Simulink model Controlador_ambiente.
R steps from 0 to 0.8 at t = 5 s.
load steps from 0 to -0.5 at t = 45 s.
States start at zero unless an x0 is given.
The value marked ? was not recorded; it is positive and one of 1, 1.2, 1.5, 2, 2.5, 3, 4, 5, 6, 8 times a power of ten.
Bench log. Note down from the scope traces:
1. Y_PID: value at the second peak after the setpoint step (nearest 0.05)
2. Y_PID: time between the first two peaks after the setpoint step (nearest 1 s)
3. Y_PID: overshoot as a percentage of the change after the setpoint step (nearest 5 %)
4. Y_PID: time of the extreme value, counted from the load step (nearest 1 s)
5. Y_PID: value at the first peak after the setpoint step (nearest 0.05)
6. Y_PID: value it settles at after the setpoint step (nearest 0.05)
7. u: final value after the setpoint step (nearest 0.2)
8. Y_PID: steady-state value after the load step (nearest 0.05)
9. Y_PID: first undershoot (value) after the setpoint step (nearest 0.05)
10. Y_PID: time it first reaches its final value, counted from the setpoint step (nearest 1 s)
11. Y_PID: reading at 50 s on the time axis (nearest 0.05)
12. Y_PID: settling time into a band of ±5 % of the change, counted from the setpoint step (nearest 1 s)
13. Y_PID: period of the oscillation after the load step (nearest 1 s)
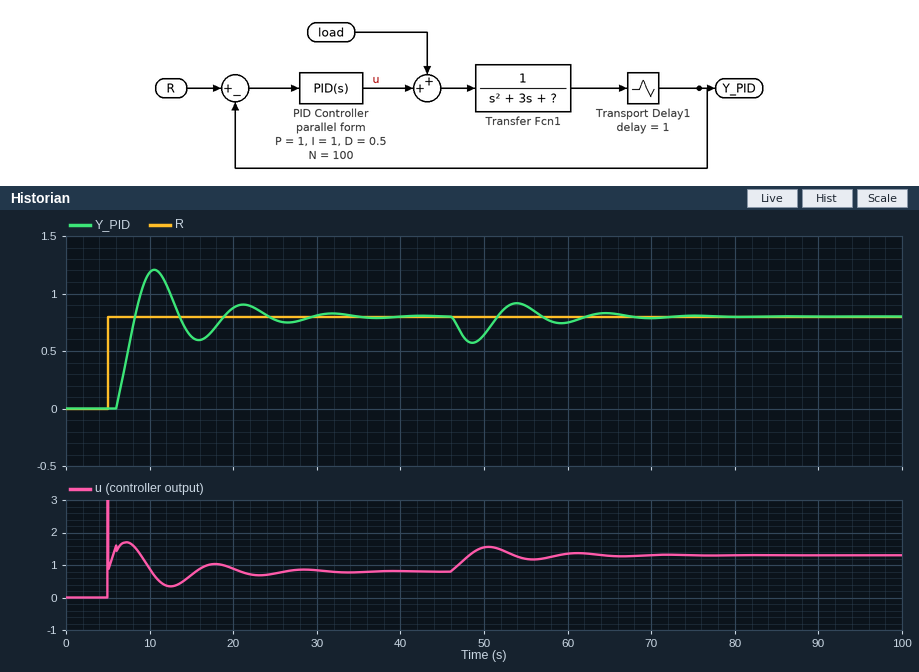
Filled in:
0.90
11 s
50 %
4 s
1.20
0.80
0.8
0.80
0.60
3 s
0.65
23 s
11 s
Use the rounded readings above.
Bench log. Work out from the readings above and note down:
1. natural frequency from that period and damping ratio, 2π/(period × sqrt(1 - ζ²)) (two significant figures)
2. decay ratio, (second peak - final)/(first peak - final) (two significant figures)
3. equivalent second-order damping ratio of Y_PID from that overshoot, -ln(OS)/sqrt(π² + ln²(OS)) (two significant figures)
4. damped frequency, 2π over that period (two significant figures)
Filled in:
0.59 rad/s
0.25
0.22
0.57 rad/s
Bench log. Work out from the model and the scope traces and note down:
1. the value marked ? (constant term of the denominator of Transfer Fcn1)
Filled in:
1
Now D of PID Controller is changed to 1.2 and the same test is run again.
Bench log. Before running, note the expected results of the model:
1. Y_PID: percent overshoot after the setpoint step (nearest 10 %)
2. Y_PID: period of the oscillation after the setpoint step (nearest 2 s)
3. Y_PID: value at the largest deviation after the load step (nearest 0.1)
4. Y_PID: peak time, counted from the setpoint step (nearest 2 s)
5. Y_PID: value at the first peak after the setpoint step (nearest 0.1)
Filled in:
30 %
12 s
0.6
6 s
1.1
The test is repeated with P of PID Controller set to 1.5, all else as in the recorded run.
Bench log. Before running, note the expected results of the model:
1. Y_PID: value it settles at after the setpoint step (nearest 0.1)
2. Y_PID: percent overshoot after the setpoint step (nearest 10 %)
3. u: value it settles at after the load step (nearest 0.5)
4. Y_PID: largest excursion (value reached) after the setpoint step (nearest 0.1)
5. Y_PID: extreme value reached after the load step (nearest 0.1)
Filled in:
0.8
40 %
1.5
1.1
0.6
